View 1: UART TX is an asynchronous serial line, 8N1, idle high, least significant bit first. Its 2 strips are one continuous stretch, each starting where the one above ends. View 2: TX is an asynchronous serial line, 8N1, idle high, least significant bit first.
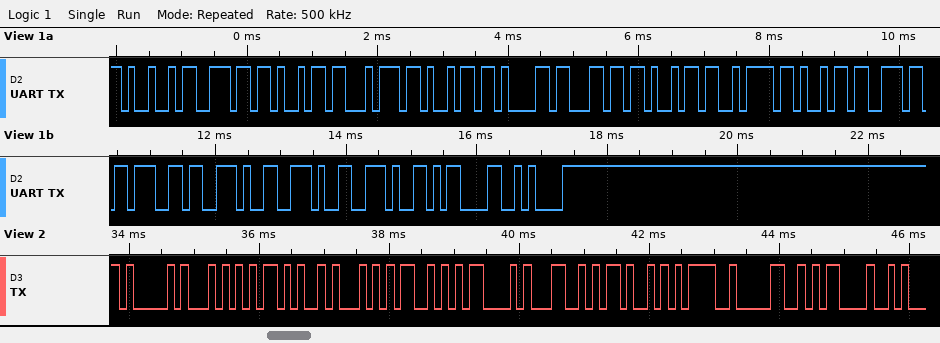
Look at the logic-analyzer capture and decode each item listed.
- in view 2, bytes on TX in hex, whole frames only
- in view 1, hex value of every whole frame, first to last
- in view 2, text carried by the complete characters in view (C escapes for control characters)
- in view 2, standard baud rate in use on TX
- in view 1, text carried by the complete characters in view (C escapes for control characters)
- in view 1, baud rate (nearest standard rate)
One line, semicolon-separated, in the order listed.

41 54 2B 51 53 43 4C 4B 3D 30 0D; 49 6E 69 74 69 61 6C 69 7A 69 6E 67 2E 2E 2E 0D 0A; "AT+QSCLK=0\r"; 9600 baud; "Initializing...\r\n"; 9600 baud
